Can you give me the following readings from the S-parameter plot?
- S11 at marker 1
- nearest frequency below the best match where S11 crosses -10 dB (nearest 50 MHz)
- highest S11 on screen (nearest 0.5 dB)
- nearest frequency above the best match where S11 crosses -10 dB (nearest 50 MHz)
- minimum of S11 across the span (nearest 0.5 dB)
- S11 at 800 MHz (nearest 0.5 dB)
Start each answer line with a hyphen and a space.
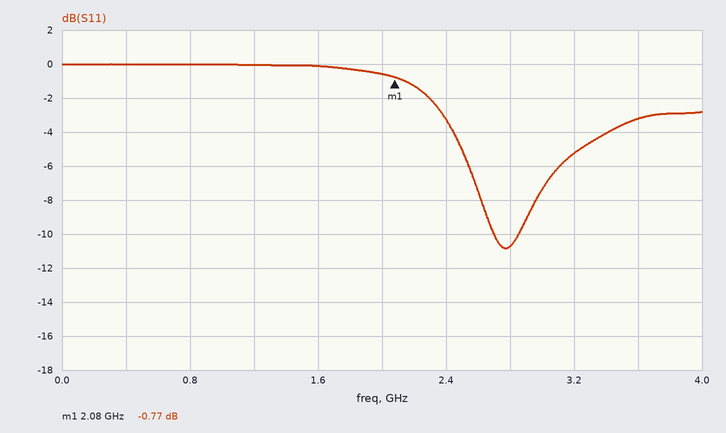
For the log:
- -0.77 dB
- 2.70 GHz
- 0.0 dB
- 2.85 GHz
- -11.0 dB
- 0.0 dB
